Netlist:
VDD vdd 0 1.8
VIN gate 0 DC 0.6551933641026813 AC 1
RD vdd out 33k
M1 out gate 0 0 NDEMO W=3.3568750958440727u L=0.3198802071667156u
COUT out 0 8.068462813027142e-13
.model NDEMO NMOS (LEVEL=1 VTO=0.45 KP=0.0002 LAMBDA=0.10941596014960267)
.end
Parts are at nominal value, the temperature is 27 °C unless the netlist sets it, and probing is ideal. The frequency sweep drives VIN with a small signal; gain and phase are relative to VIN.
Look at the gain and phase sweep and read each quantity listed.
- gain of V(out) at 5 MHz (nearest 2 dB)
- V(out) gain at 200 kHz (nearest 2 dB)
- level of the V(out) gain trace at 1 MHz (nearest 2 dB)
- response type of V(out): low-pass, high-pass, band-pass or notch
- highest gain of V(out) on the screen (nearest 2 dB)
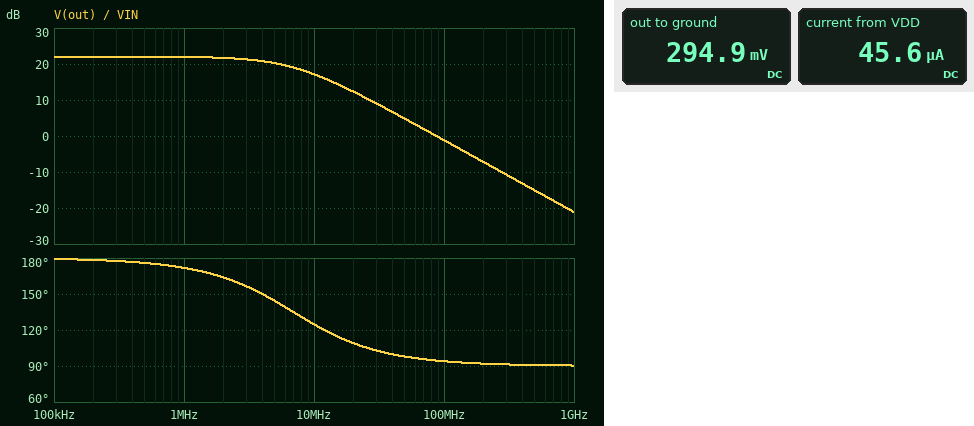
20 dB
22 dB
22 dB
low-pass
22 dB
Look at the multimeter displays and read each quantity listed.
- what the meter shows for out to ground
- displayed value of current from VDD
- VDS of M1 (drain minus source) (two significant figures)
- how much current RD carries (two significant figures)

294.9 mV
45.6 µA
290 mV
46 µA
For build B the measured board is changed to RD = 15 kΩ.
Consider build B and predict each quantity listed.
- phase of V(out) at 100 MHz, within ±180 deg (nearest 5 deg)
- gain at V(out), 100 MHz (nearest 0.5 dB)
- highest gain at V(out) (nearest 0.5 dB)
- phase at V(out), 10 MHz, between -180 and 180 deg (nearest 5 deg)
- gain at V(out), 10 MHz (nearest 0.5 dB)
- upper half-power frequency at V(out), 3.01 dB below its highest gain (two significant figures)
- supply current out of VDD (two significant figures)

100 deg
-0.5 dB
16.5 dB
145 deg
15.0 dB
14 MHz
49 µA
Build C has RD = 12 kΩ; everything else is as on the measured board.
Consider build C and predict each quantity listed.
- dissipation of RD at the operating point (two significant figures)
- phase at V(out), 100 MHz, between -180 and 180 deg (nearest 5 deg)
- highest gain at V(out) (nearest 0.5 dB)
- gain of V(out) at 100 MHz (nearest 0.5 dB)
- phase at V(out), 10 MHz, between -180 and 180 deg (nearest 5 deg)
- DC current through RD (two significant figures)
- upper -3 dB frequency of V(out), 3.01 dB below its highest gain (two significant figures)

30 µW
100 deg
15.0 dB
-0.5 dB
150 deg
50 µA
17 MHz
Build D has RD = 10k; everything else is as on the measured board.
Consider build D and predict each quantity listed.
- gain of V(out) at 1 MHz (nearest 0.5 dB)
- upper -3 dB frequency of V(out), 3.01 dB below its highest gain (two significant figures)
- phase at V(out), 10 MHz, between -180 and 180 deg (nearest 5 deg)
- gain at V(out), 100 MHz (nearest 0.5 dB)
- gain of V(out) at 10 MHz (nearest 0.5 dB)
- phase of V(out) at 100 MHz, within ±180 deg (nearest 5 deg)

13.5 dB
21 MHz
155 deg
-0.5 dB
12.5 dB
100 deg
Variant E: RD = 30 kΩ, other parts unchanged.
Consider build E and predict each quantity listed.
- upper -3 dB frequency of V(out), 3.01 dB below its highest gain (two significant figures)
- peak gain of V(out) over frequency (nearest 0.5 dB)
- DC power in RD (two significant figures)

7.5 MHz
21.5 dB
64 µW
